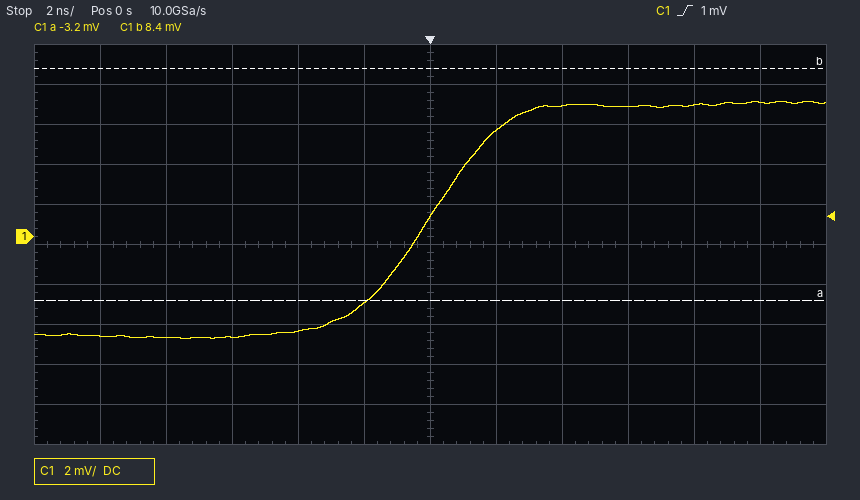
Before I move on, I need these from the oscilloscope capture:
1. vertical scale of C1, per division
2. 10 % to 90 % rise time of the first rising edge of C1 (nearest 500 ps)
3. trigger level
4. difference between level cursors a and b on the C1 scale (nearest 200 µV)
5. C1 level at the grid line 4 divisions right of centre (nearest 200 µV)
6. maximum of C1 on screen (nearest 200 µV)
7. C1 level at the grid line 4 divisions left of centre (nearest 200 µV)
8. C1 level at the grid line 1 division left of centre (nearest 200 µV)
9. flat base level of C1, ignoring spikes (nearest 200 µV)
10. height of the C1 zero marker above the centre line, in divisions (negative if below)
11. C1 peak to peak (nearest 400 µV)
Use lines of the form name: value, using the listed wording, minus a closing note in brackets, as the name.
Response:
vertical scale of C1, per division: 2 mV
10 % to 90 % rise time of the first rising edge of C1: 4.5 ns
trigger level: 1 mV
difference between level cursors a and b on the C1 scale: 11.6 mV
C1 level at the grid line 4 divisions right of centre: 6.6 mV
maximum of C1 on screen: 6.8 mV
C1 level at the grid line 4 divisions left of centre: -5.0 mV
C1 level at the grid line 1 division left of centre: -3.4 mV
flat base level of C1, ignoring spikes: -5.0 mV
height of the C1 zero marker above the centre line, in divisions: +0.2 div
C1 peak to peak: 12.0 mV
